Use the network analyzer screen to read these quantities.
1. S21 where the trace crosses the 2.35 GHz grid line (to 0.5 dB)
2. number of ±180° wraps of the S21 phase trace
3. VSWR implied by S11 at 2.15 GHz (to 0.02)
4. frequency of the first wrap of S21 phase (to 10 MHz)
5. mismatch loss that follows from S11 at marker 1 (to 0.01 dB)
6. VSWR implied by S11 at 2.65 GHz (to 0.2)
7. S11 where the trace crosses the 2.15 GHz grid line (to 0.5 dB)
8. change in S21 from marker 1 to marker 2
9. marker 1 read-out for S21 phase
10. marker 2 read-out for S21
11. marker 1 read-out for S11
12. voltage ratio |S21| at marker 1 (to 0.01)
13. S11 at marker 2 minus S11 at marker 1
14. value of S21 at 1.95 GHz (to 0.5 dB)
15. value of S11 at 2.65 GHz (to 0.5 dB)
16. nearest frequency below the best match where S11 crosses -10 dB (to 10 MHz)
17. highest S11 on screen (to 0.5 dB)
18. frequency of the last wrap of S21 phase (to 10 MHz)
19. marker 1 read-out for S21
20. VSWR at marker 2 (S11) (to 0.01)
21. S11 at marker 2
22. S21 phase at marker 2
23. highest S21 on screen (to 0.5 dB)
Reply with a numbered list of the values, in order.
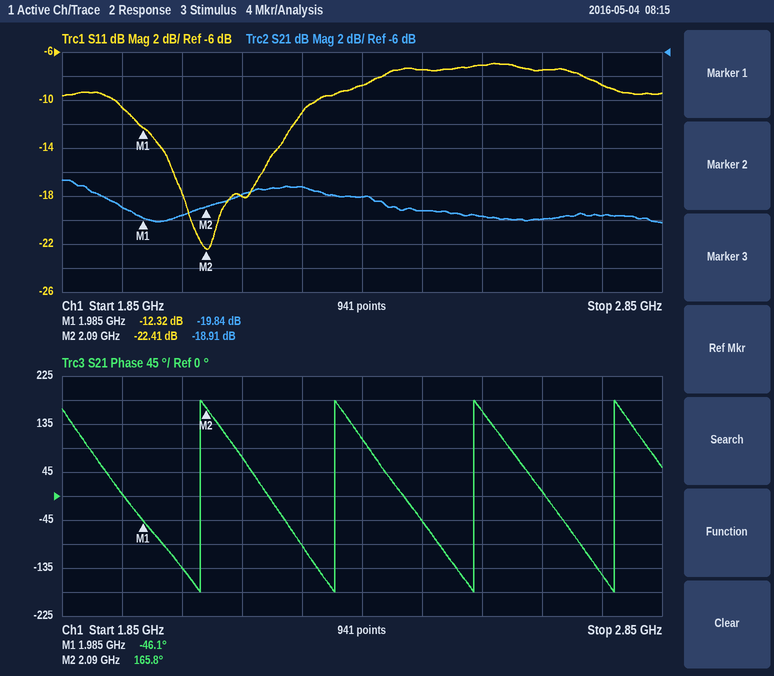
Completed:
1. -18.0 dB
2. 4
3. 1.28
4. 2.08 GHz
5. 0.26 dB
6. 2.4
7. -18.0 dB
8. 0.93 dB
9. -46.1°
10. -18.91 dB
11. -12.32 dB
12. 0.10
13. -10.09 dB
14. -19.0 dB
15. -7.5 dB
16. 1.94 GHz
17. -7.0 dB
18. 2.77 GHz
19. -19.84 dB
20. 1.16
21. -22.41 dB
22. 165.8°
23. -16.5 dB
